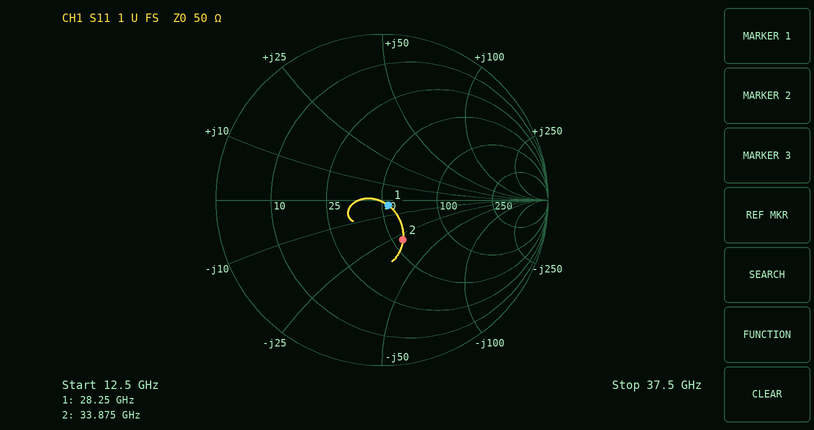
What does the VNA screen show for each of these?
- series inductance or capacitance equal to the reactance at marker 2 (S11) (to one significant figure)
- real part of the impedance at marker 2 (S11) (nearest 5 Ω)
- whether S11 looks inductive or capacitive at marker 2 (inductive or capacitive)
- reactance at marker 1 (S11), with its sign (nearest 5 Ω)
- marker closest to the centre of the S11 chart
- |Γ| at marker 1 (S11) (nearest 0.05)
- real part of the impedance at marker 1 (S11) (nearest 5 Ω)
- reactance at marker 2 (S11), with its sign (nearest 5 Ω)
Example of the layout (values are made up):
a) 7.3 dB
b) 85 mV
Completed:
a) 200 fF
b) 55 Ω
c) capacitive
d) -5 Ω
e) marker 1
f) 0.05
g) 55 Ω
h) -30 Ω
